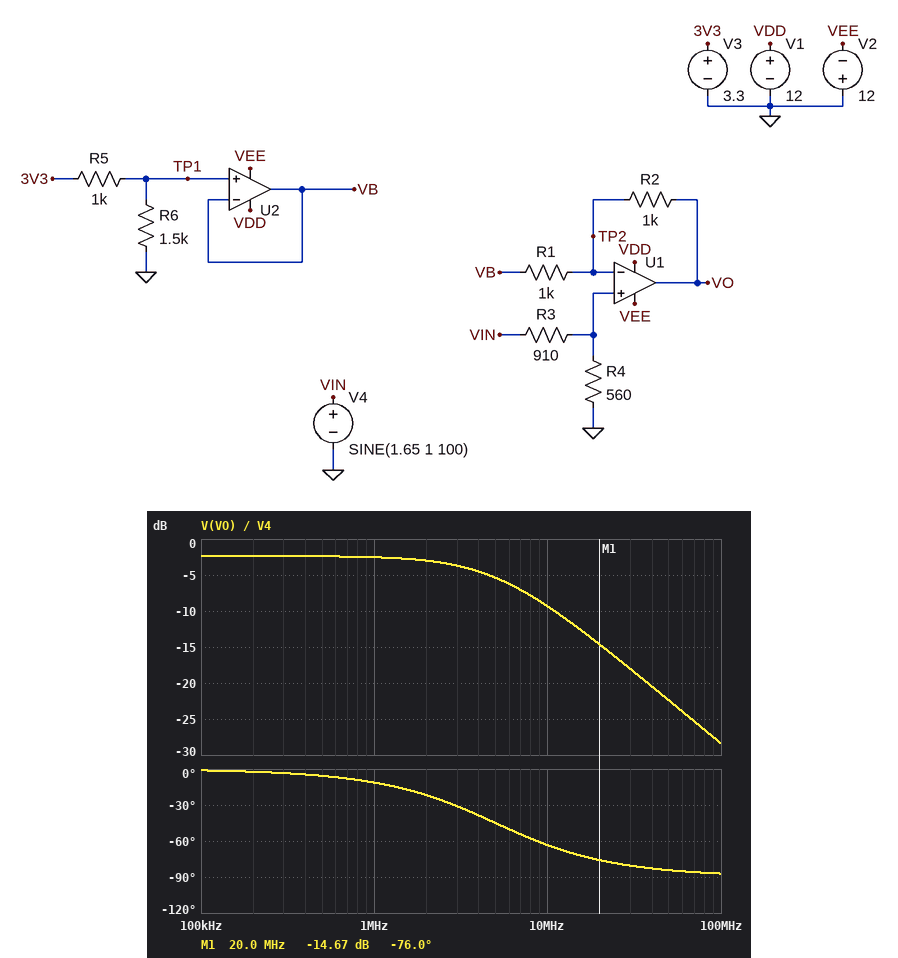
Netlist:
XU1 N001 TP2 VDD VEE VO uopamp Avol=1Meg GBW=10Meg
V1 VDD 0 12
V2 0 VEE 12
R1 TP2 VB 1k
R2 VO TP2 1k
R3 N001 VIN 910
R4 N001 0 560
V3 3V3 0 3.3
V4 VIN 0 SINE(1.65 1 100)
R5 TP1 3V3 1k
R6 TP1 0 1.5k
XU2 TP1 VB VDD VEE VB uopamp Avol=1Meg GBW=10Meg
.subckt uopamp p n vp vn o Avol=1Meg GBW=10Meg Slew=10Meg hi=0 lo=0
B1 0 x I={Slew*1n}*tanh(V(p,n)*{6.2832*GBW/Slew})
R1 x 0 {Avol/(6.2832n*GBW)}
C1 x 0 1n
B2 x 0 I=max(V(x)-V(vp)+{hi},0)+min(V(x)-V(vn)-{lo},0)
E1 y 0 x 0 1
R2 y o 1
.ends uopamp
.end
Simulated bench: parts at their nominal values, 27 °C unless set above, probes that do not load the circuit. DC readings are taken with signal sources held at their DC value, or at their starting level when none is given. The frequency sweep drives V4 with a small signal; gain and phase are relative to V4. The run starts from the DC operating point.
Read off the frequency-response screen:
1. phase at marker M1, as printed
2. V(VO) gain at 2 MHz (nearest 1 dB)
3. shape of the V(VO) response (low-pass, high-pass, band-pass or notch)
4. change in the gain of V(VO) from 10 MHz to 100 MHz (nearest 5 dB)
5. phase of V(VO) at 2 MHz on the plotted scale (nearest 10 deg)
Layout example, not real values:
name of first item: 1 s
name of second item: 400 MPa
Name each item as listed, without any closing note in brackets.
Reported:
phase at marker M1, as printed: -76.0 deg
V(VO) gain at 2 MHz: -3 dB
shape of the V(VO) response: low-pass
change in the gain of V(VO) from 10 MHz to 100 MHz: -20 dB
phase of V(VO) at 2 MHz on the plotted scale: -20 deg
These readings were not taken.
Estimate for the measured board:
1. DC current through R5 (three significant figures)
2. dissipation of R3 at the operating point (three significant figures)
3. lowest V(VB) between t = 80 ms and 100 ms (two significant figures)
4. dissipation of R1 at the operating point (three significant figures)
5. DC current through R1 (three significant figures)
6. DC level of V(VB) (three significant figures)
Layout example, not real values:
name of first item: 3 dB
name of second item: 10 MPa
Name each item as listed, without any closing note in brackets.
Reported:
DC current through R5: 1.32 mA
dissipation of R3 at the operating point: 1.15 mW
lowest V(VB) between t = 80 ms and 100 ms: 2.0 V
dissipation of R1 at the operating point: 1.83 mW
DC current through R1: 1.35 mA
DC level of V(VB): 1.98 V
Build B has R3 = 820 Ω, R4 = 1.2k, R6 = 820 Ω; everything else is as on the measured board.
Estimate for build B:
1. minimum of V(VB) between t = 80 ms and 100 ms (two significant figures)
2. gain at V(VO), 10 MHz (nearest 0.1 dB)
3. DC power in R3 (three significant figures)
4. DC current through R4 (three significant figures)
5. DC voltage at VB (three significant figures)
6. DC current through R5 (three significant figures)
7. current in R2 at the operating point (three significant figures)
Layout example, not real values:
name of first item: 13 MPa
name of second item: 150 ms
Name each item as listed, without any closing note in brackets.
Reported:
minimum of V(VB) between t = 80 ms and 100 ms: 1.5 V
gain at V(VO), 10 MHz: -5.5 dB
DC power in R3: 547 µW
DC current through R4: 817 µA
DC voltage at VB: 1.49 V
DC current through R5: 1.81 mA
current in R2 at the operating point: 507 µA
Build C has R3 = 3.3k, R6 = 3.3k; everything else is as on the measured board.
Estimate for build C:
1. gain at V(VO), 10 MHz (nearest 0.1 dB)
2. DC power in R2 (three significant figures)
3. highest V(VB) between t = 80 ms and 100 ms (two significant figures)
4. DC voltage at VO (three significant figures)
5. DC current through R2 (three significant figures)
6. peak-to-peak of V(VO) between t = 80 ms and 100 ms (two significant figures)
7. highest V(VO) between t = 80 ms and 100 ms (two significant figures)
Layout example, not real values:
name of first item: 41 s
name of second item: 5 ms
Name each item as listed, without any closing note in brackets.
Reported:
gain at V(VO), 10 MHz: -17.7 dB
DC power in R2: 5.26 mW
highest V(VB) between t = 80 ms and 100 ms: 2.5 V
DC voltage at VO: -2.05 V
DC current through R2: 2.29 mA
peak-to-peak of V(VO) between t = 80 ms and 100 ms: 580 mV
highest V(VO) between t = 80 ms and 100 ms: -1.8 V
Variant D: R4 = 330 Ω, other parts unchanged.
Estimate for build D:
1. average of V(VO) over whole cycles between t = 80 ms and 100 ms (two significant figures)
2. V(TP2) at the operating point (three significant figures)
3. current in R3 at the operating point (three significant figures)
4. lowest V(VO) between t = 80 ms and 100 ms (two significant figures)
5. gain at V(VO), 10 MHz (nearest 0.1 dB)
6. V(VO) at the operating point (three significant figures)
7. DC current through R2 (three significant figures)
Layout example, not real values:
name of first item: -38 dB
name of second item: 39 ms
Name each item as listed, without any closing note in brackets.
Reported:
average of V(VO) over whole cycles between t = 80 ms and 100 ms: -1.1 V
V(TP2) at the operating point: 439 mV
current in R3 at the operating point: 1.33 mA
lowest V(VO) between t = 80 ms and 100 ms: -1.6 V
gain at V(VO), 10 MHz: -12.5 dB
V(VO) at the operating point: -1.10 V
DC current through R2: 1.54 mA
